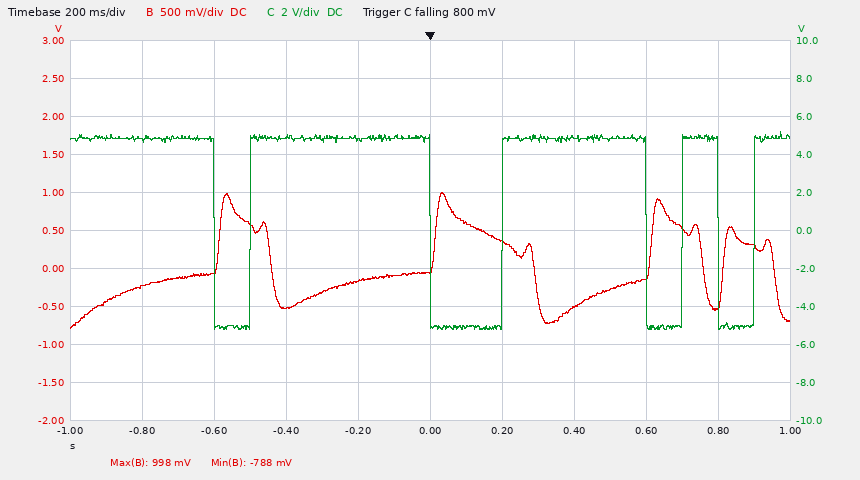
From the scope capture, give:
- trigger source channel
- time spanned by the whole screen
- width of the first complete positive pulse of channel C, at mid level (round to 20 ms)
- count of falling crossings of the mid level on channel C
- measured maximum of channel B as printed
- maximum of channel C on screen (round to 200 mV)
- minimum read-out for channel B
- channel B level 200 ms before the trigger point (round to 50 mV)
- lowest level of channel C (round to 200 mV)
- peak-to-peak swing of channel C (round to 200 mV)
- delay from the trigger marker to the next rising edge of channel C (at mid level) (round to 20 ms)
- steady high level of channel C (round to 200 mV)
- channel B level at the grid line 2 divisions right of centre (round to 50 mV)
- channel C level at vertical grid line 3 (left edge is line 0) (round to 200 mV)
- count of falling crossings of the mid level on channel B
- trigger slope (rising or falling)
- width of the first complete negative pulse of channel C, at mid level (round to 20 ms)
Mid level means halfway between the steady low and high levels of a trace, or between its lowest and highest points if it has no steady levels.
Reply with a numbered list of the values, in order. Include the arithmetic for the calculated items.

1. channel C
2. 2 s
3. 500 ms
4. 4
5. 998 mV
6. 5.2 V
7. -788 mV
8. -150 mV
9. -5.2 V
10. 5.2 V − (-5.2 V) = 10.4 V
11. 200 ms
12. 4.8 V
13. -500 mV
14. 5.0 V
15. 4
16. falling
17. 100 ms
